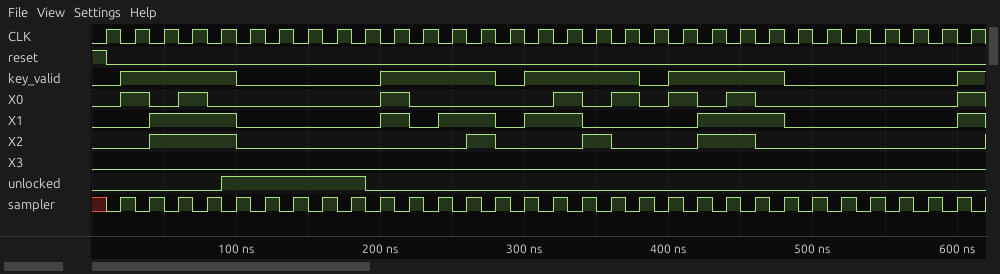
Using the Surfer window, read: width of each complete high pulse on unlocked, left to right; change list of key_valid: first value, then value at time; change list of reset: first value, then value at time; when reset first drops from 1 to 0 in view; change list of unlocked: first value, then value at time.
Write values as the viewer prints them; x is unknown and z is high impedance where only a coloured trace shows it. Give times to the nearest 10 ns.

100 ns
0, 1 at 20 ns, 0 at 100 ns, 1 at 200 ns, 0 at 280 ns, 1 at 300 ns, 0 at 380 ns, 1 at 400 ns, 0 at 480 ns, 1 at 600 ns
1, 0 at 10 ns
10 ns
0, 1 at 90 ns, 0 at 190 ns
